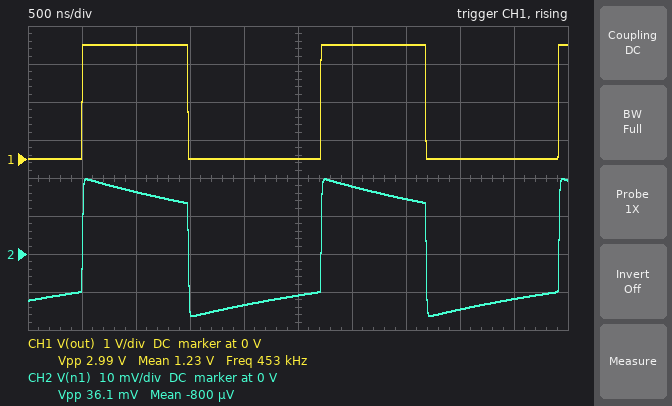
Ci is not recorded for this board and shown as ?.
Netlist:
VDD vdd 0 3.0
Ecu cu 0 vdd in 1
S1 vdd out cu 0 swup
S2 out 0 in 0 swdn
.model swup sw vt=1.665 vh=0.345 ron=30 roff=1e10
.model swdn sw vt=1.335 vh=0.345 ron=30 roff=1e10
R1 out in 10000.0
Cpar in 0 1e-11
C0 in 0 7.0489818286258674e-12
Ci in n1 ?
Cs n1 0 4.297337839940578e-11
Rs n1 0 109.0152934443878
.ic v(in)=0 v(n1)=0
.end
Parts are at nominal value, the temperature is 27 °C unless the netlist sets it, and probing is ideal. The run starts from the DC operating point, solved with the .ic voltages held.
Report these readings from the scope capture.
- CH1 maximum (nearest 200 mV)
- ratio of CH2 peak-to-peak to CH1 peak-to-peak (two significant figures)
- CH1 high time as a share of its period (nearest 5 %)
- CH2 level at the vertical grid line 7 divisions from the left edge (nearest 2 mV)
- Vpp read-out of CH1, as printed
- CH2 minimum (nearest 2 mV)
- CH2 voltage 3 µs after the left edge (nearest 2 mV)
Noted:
3.0 V
0.012
45 %
14 mV
2.99 V
-16 mV
18 mV
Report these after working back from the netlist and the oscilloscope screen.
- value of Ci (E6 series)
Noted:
220 pF
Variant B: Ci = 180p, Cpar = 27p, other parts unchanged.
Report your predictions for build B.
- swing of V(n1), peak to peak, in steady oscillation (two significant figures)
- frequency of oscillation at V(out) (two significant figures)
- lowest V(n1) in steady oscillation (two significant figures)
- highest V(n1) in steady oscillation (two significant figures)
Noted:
33 mV
500 kHz
-15 mV
18 mV
